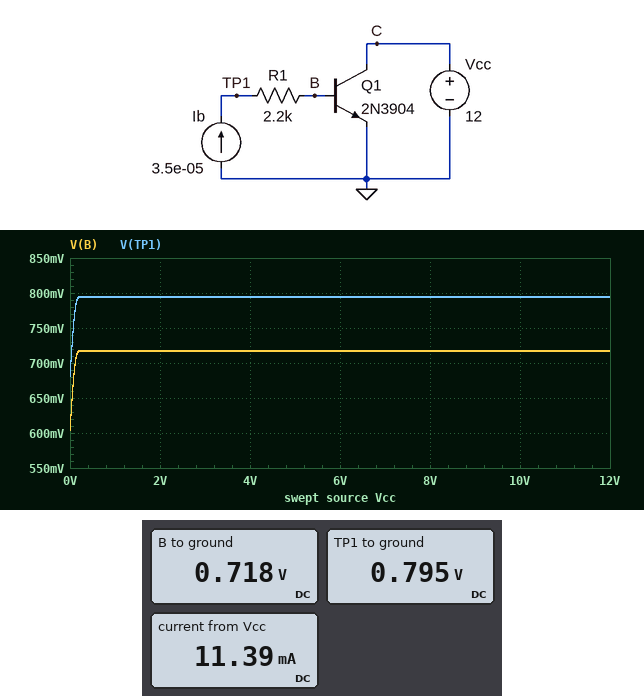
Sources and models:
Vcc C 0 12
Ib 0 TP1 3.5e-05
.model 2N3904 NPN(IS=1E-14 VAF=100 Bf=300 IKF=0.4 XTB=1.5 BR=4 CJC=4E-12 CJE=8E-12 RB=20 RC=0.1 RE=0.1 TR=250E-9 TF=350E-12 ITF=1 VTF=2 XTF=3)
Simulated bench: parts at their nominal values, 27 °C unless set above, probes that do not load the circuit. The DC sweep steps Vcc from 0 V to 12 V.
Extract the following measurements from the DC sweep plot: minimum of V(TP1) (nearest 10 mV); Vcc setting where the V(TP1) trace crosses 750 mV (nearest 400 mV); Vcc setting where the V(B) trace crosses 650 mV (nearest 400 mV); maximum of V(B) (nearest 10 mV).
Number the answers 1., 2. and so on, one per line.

1. 680 mV
2. 0 V
3. 0 V
4. 720 mV
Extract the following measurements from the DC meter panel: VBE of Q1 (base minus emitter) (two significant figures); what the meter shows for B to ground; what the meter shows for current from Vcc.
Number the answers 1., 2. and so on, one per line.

1. 720 mV
2. 0.718 V
3. 11.39 mA
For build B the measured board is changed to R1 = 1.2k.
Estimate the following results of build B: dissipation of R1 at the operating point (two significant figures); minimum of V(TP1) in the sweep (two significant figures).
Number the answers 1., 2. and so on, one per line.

1. 1.5 µW
2. 650 mV
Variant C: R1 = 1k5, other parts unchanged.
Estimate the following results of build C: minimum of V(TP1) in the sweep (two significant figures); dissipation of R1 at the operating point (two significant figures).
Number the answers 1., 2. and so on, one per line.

1. 660 mV
2. 1.8 µW
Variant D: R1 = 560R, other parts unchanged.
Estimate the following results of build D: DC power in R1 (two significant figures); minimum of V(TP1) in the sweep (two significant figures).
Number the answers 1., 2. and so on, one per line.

1. 690 nW
2. 620 mV
